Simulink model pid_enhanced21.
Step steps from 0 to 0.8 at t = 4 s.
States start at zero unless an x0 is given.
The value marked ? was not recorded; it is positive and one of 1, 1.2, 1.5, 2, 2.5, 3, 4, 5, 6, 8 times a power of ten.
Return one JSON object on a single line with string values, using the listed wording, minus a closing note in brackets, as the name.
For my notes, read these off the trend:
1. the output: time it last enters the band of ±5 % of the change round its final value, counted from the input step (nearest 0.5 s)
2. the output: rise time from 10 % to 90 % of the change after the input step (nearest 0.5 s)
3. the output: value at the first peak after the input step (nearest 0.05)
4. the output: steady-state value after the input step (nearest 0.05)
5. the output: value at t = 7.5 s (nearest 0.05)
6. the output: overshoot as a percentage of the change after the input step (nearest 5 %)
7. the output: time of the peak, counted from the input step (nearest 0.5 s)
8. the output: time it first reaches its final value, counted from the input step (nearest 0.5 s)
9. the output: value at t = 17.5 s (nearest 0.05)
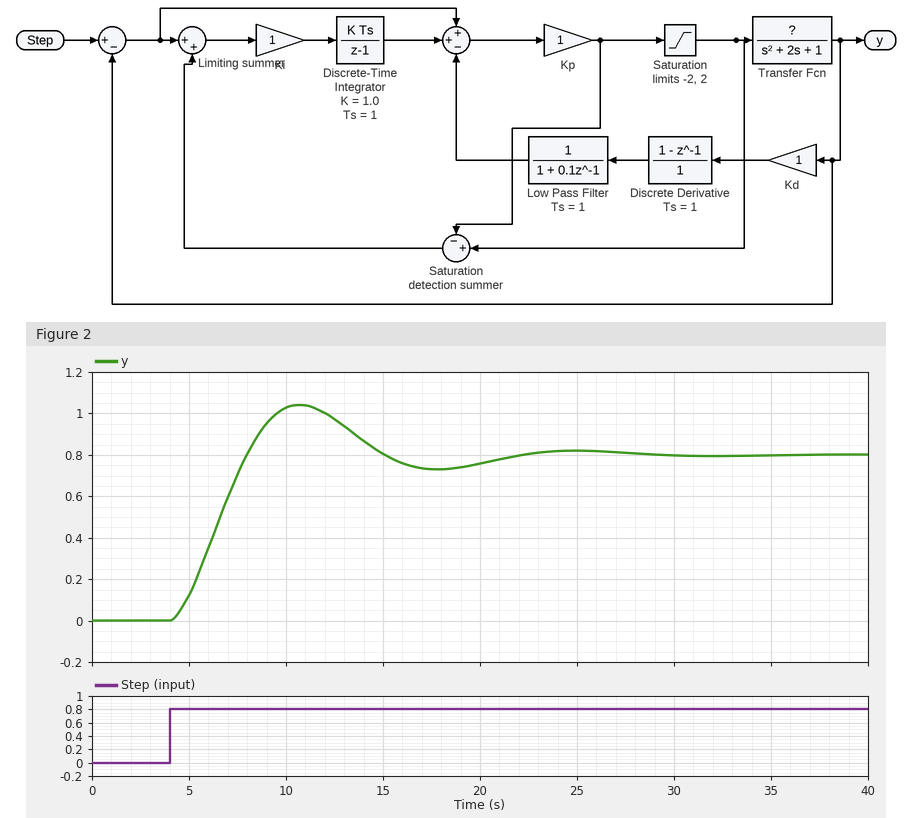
{"the output: time it last enters the band of ±5 % of the change round its final value, counted from the input step": "16.0 s", "the output: rise time from 10 % to 90 % of the change after the input step": "3.0 s", "the output: value at the first peak after the input step": "1.05", "the output: steady-state value after the input step": "0.80", "the output: value at t = 7.5 s": "0.70", "the output: overshoot as a percentage of the change after the input step": "30 %", "the output: time of the peak, counted from the input step": "6.5 s", "the output: time it first reaches its final value, counted from the input step": "4.0 s", "the output: value at t = 17.5 s": "0.75"}
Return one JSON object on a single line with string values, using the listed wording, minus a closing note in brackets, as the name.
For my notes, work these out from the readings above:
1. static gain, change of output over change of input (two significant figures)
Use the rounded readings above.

{"static gain, change of output over change of input": "1.0"}
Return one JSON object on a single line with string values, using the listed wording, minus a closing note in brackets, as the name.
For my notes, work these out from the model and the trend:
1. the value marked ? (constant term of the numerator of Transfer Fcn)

{"the value marked ?": "0.6"}
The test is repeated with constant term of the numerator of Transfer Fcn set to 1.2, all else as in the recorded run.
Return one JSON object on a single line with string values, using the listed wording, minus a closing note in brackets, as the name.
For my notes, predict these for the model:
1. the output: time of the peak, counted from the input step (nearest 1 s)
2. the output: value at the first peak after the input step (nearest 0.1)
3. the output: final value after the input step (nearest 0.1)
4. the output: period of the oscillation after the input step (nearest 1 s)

{"the output: time of the peak, counted from the input step": "5 s", "the output: value at the first peak after the input step": "1.2", "the output: final value after the input step": "0.8", "the output: period of the oscillation after the input step": "11 s"}
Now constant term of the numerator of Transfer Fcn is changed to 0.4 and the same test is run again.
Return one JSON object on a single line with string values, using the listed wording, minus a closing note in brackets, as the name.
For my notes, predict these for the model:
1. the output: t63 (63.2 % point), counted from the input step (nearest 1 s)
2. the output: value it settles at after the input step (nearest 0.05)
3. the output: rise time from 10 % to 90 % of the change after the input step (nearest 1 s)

{"the output: t63 (63.2 % point), counted from the input step": "3 s", "the output: value it settles at after the input step": "0.80", "the output: rise time from 10 % to 90 % of the change after the input step": "4 s"}
